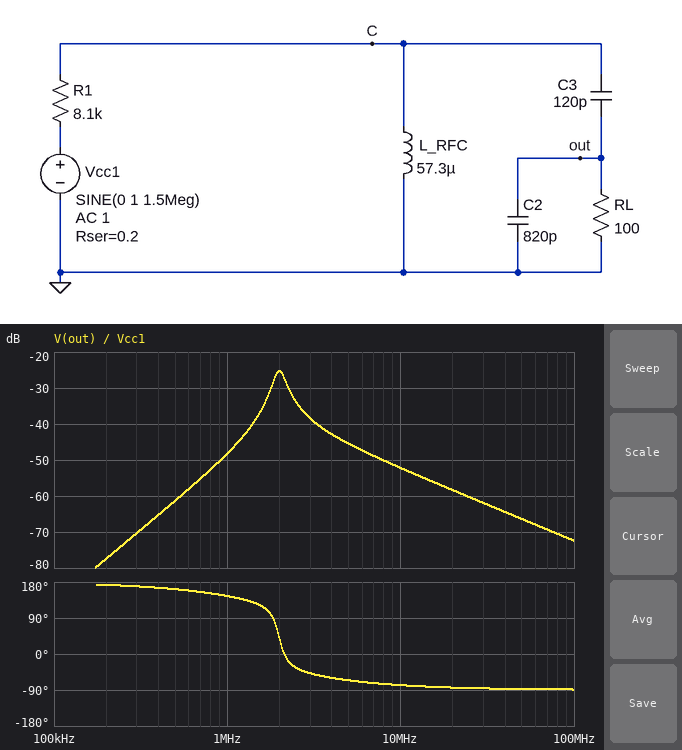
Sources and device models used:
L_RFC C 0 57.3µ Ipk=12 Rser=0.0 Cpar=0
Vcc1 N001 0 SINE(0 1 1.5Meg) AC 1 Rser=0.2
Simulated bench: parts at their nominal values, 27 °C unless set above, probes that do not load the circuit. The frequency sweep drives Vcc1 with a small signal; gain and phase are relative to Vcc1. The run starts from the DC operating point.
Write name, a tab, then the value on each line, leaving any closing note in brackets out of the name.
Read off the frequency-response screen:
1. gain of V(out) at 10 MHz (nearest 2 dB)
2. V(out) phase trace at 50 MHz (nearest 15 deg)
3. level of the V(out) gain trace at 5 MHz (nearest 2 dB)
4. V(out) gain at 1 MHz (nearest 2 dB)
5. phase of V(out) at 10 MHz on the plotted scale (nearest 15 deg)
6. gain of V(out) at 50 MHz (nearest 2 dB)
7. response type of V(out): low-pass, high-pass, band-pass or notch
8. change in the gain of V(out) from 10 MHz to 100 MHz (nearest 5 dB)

gain of V(out) at 10 MHz	-52 dB
V(out) phase trace at 50 MHz	-90 deg
level of the V(out) gain trace at 5 MHz	-46 dB
V(out) gain at 1 MHz	-48 dB
phase of V(out) at 10 MHz on the plotted scale	-75 deg
gain of V(out) at 50 MHz	-66 dB
response type of V(out): low-pass, high-pass, band-pass or notch	band-pass
change in the gain of V(out) from 10 MHz to 100 MHz	-20 dB
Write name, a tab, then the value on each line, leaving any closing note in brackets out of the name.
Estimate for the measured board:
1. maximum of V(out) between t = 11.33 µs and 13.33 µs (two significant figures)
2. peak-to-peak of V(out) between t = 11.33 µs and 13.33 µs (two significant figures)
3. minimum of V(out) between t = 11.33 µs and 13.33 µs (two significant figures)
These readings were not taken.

maximum of V(out) between t = 11.33 µs and 13.33 µs	13 mV
peak-to-peak of V(out) between t = 11.33 µs and 13.33 µs	26 mV
minimum of V(out) between t = 11.33 µs and 13.33 µs	-13 mV
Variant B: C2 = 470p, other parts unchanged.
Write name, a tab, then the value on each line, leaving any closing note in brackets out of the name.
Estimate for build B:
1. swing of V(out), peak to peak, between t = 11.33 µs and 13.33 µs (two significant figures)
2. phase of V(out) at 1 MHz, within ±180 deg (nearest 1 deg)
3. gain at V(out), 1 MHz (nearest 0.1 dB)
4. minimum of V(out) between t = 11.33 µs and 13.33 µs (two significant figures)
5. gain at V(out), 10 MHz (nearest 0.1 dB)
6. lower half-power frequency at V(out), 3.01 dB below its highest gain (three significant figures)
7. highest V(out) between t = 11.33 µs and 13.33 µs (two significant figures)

swing of V(out), peak to peak, between t = 11.33 µs and 13.33 µs	30 mV
phase of V(out) at 1 MHz, within ±180 deg	155 deg
gain at V(out), 1 MHz	-47.4 dB
minimum of V(out) between t = 11.33 µs and 13.33 µs	-15 mV
gain at V(out), 10 MHz	-47.7 dB
lower half-power frequency at V(out), 3.01 dB below its highest gain	1.81 MHz
highest V(out) between t = 11.33 µs and 13.33 µs	15 mV
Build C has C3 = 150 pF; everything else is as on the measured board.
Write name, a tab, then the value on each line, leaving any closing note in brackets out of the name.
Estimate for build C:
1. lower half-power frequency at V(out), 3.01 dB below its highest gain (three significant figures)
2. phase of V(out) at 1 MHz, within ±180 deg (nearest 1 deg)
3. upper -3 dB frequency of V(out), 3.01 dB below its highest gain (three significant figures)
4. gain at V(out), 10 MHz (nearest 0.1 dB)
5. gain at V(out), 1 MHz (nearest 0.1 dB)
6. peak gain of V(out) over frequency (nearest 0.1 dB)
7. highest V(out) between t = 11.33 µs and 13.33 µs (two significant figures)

lower half-power frequency at V(out), 3.01 dB below its highest gain	1.65 MHz
phase of V(out) at 1 MHz, within ±180 deg	143 deg
upper -3 dB frequency of V(out), 3.01 dB below its highest gain	1.96 MHz
gain at V(out), 10 MHz	-52.3 dB
gain at V(out), 1 MHz	-45.6 dB
peak gain of V(out) over frequency	-25.1 dB
highest V(out) between t = 11.33 µs and 13.33 µs	22 mV
